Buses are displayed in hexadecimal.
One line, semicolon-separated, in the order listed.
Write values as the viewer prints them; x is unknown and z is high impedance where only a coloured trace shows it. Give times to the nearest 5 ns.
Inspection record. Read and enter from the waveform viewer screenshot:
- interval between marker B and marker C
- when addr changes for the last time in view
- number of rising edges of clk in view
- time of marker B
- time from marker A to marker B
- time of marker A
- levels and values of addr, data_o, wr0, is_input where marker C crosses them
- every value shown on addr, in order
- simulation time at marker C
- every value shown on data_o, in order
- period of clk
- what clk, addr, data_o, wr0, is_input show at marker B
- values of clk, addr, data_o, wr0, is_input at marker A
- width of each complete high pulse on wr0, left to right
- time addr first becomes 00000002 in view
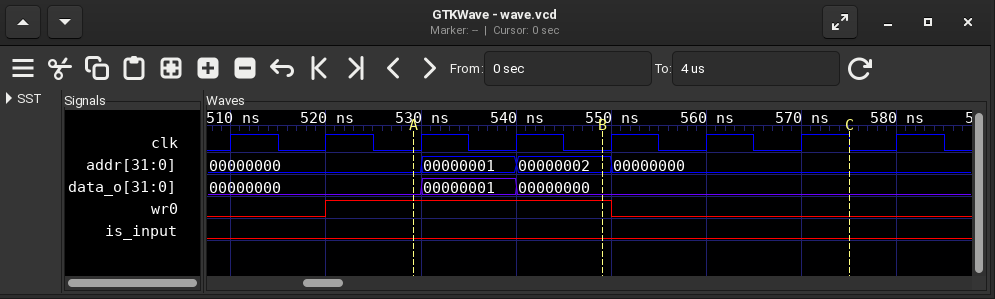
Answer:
25 ns; 550 ns; 8; 550 ns; 20 ns; 530 ns; addr=00000000, data_o=00000000, wr0=0, is_input=0; 00000000, 00000001, 00000002, 00000000; 575 ns; 00000000, 00000001, 00000000; 10 ns; clk=0, addr=00000002, data_o=00000000, wr0=1, is_input=0; clk=0, addr=00000000, data_o=00000000, wr0=1, is_input=0; 30 ns; 540 ns
